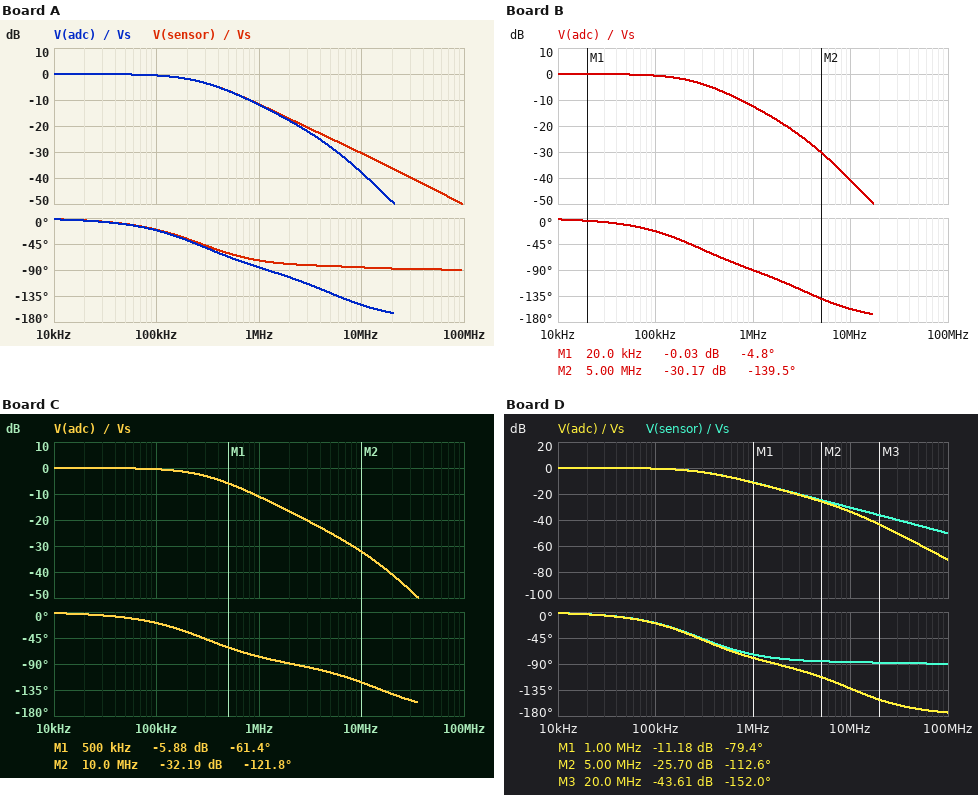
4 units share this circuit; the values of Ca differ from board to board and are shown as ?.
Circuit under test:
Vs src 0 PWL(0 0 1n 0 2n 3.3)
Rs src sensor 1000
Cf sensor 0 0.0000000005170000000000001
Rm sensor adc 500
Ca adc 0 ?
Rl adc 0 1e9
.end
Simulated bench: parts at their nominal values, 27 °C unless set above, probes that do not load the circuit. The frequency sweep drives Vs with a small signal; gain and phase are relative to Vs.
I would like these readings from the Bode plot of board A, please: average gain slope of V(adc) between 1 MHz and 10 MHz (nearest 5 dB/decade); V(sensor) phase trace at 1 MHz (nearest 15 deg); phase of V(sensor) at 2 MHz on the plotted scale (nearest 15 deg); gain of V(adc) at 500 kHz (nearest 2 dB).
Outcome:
-25 dB/decade
-75 deg
-75 deg
-6 dB
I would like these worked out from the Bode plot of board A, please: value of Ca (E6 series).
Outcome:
68 pF
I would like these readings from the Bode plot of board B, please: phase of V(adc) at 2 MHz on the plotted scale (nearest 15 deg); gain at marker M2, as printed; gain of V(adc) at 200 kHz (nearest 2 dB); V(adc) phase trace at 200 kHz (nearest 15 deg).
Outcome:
-105 deg
-30.17 dB
-2 dB
-45 deg
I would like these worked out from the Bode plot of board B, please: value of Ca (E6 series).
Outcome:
100 pF
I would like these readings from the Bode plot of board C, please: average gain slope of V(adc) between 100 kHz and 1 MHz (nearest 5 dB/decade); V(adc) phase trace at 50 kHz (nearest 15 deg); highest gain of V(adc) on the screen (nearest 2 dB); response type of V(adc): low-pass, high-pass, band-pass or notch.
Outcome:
-10 dB/decade
-15 deg
0 dB
low-pass
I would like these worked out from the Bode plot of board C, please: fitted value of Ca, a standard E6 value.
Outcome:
22 pF
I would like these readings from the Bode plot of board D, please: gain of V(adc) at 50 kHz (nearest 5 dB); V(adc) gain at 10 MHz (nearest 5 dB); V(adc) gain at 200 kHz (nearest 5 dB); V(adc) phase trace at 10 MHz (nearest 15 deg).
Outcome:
0 dB
-35 dB
0 dB
-135 deg
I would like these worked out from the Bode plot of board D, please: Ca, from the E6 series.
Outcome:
33 pF
